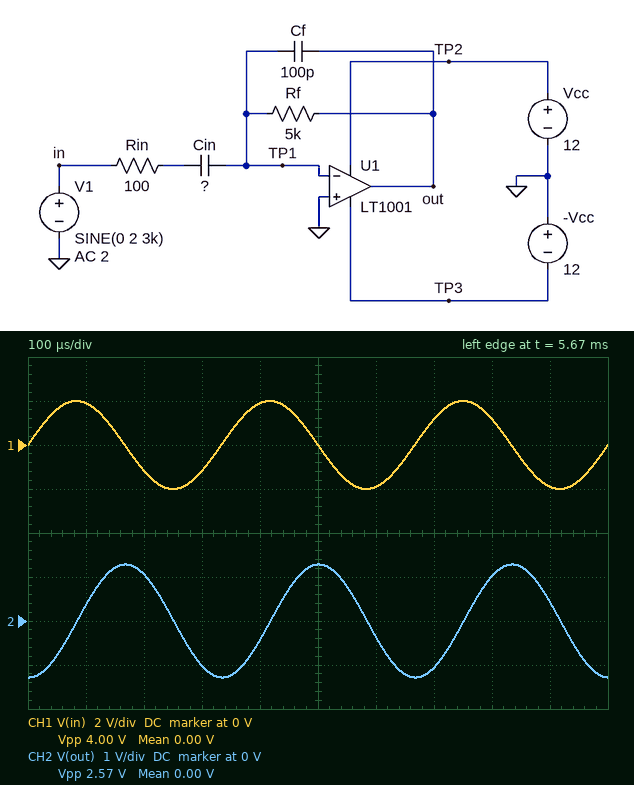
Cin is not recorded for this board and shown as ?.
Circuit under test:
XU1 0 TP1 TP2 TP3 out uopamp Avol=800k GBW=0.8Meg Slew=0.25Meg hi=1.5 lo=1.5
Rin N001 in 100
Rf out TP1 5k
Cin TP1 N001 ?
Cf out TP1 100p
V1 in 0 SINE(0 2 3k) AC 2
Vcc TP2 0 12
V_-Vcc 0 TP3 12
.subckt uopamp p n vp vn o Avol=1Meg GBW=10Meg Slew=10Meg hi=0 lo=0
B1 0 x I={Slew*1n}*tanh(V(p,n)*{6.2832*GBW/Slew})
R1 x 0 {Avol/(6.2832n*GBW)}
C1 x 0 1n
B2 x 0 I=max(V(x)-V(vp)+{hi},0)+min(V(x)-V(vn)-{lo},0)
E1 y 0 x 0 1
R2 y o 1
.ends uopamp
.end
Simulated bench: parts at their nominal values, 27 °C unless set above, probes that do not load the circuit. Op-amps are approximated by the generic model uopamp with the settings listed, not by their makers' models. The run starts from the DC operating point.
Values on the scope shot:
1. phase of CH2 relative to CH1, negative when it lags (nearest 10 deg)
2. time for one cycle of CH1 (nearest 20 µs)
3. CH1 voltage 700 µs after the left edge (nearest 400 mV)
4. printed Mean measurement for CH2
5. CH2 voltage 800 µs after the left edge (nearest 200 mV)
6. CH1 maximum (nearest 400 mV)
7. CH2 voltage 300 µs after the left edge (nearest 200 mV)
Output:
-90 deg
340 µs
1.2 V
0.00 V
1.0 V
2.0 V
-1.0 V
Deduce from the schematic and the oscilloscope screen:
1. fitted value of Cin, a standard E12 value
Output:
6.8 nF
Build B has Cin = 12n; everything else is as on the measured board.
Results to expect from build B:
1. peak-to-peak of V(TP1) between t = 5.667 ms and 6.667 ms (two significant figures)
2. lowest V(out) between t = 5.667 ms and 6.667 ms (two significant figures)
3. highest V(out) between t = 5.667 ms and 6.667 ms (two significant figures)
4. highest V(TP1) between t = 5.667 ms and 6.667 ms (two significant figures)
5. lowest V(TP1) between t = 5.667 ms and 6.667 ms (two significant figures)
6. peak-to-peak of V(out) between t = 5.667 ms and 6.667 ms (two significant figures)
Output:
17 mV
-2.3 V
2.3 V
8.6 mV
-8.6 mV
4.5 V
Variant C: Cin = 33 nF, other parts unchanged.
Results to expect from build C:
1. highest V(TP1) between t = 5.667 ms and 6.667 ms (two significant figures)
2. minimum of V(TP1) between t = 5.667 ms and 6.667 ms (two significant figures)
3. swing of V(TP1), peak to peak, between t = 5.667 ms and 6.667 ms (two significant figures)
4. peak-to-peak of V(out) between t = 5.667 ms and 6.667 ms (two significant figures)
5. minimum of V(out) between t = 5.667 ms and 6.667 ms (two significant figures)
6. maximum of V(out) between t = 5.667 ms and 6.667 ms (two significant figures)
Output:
26 mV
-26 mV
51 mV
13 V
-6.3 V
6.3 V
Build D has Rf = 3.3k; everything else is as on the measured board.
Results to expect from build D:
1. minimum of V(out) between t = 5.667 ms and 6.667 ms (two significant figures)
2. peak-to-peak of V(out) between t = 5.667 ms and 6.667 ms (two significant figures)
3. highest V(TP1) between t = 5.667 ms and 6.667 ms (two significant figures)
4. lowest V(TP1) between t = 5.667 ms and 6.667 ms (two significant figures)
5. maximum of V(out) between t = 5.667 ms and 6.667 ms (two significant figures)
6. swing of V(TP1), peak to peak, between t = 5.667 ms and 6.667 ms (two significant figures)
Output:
-850 mV
1.7 V
3.2 mV
-3.2 mV
850 mV
6.4 mV
